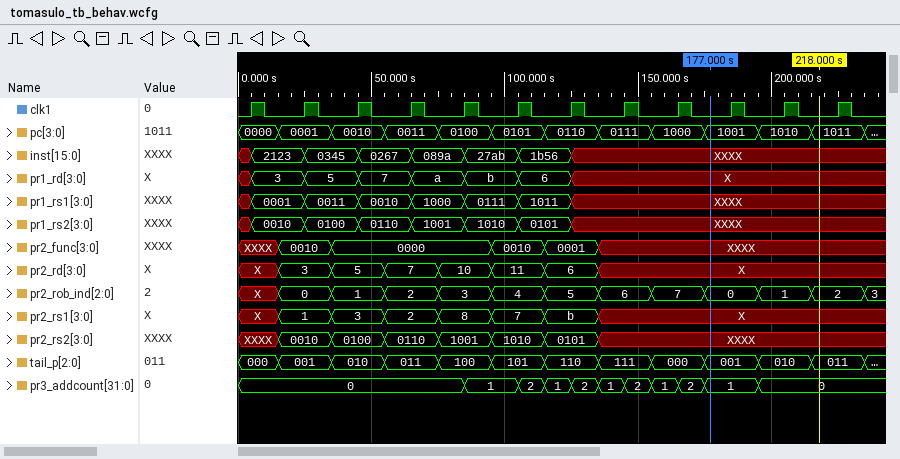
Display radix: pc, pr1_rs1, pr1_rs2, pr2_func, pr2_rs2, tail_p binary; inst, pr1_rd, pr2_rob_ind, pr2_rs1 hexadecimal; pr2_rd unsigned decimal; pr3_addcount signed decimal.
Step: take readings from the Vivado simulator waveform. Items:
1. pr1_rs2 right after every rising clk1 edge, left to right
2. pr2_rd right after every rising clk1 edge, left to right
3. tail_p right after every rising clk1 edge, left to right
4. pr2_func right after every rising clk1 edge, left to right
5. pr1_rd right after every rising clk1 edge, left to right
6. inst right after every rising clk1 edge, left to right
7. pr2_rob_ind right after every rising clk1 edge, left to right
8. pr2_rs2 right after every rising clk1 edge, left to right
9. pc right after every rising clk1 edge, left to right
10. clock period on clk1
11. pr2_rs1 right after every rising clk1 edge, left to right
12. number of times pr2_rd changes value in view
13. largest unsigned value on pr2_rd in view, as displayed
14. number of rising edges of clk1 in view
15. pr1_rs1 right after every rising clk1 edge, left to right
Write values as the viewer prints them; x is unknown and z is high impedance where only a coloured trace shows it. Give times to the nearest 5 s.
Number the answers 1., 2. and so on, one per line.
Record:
1. 0010, 0100, 0110, 1001, 1010, 0101, XXXX, XXXX, XXXX, XXXX, XXXX, XXXX
2. X, 3, 5, 7, 10, 11, 6, X, X, X, X, X
3. 000, 001, 010, 011, 100, 101, 110, 111, 000, 001, 010, 011
4. XXXX, 0010, 0000, 0000, 0000, 0010, 0001, XXXX, XXXX, XXXX, XXXX, XXXX
5. 3, 5, 7, a, b, 6, X, X, X, X, X, X
6. 2123, 0345, 0267, 089a, 27ab, 1b56, XXXX, XXXX, XXXX, XXXX, XXXX, XXXX
7. X, 0, 1, 2, 3, 4, 5, 6, 7, 0, 1, 2
8. XXXX, 0010, 0100, 0110, 1001, 1010, 0101, XXXX, XXXX, XXXX, XXXX, XXXX
9. 0000, 0001, 0010, 0011, 0100, 0101, 0110, 0111, 1000, 1001, 1010, 1011
10. 20 s
11. X, 1, 3, 2, 8, 7, b, X, X, X, X, X
12. 7
13. 11
14. 12
15. 0001, 0011, 0010, 1000, 0111, 1011, XXXX, XXXX, XXXX, XXXX, XXXX, XXXX
